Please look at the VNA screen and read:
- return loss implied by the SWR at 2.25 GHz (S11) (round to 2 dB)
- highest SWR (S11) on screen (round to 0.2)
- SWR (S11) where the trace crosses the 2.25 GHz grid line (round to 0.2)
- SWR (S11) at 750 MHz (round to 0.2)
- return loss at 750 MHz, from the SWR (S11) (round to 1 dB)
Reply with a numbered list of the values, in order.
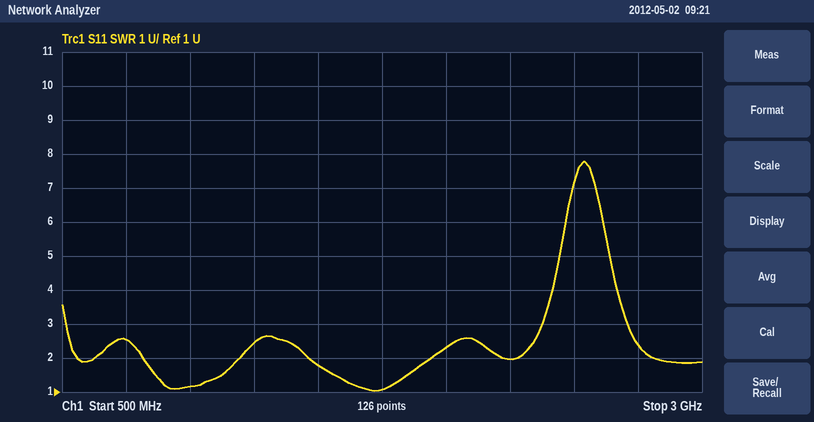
1. 10 dB
2. 7.8
3. 2.0
4. 2.6
5. 7 dB
